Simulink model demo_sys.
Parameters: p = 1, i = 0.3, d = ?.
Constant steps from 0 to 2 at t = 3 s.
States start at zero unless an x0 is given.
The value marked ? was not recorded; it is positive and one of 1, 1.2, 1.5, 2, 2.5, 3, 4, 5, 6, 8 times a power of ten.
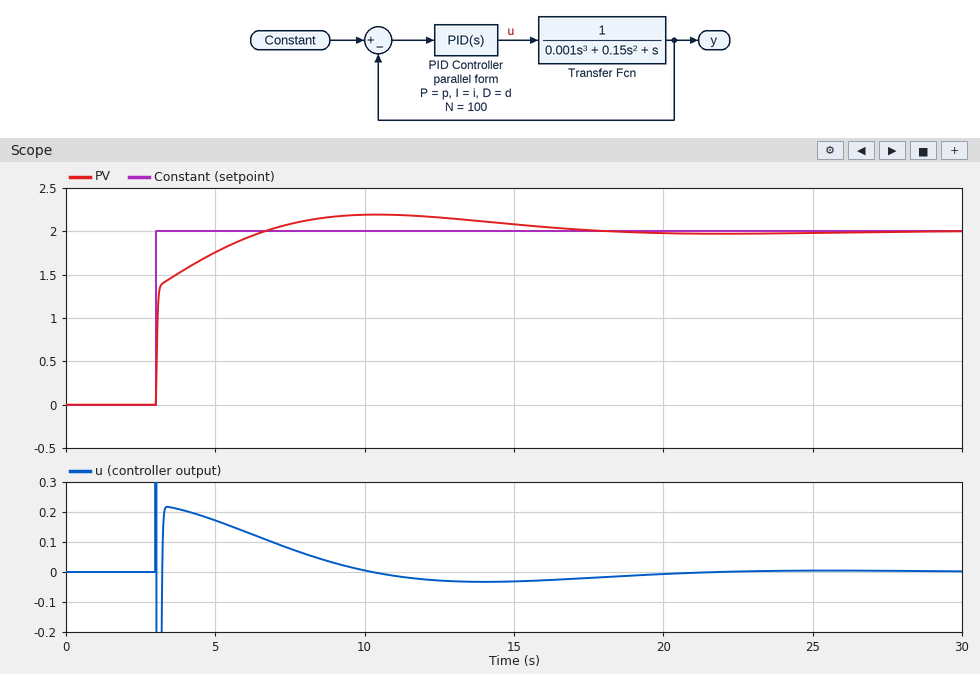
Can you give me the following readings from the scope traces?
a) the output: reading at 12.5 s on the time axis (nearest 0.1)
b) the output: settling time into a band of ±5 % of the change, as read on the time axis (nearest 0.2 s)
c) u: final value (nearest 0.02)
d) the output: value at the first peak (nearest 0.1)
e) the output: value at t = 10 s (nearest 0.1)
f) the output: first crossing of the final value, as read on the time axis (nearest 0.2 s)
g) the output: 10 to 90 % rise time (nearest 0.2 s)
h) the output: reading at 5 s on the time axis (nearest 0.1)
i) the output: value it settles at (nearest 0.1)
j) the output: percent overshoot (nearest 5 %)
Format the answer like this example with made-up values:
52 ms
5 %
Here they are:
2.2
14.4 s
0.00
2.2
2.2
6.6 s
2.2 s
1.8
2.0
10 %
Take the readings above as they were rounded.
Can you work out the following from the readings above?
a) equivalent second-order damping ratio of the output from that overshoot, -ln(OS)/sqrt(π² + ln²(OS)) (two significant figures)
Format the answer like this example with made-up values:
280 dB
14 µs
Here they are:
0.59
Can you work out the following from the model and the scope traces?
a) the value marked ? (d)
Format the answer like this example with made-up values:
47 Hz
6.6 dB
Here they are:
2
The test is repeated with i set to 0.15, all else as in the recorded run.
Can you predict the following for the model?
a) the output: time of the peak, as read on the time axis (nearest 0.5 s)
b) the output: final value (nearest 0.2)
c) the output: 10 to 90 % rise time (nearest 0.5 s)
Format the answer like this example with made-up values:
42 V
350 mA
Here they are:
12.5 s
2.0
2.5 s
